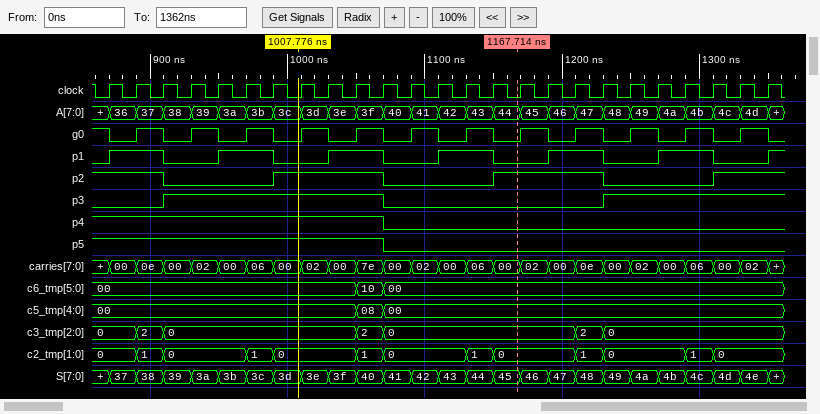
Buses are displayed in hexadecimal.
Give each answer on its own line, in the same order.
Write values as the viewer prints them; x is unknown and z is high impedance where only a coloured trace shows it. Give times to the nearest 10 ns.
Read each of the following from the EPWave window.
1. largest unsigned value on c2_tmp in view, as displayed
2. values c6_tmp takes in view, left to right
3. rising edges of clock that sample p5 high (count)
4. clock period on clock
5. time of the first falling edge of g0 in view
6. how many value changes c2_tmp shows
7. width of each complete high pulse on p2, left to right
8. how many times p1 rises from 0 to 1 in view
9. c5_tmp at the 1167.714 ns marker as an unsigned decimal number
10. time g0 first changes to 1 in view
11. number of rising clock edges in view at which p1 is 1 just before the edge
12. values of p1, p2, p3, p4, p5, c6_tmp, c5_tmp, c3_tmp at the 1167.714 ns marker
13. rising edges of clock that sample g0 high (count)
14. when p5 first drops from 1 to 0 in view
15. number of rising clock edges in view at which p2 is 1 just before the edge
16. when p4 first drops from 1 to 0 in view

1
00, 10, 00
11
20 ns
870 ns
12
80 ns, 80 ns
7
0
890 ns
12
p1=0, p2=1, p3=0, p4=0, p5=0, c6_tmp=00, c5_tmp=00, c3_tmp=0
13
1070 ns
13
1070 ns
